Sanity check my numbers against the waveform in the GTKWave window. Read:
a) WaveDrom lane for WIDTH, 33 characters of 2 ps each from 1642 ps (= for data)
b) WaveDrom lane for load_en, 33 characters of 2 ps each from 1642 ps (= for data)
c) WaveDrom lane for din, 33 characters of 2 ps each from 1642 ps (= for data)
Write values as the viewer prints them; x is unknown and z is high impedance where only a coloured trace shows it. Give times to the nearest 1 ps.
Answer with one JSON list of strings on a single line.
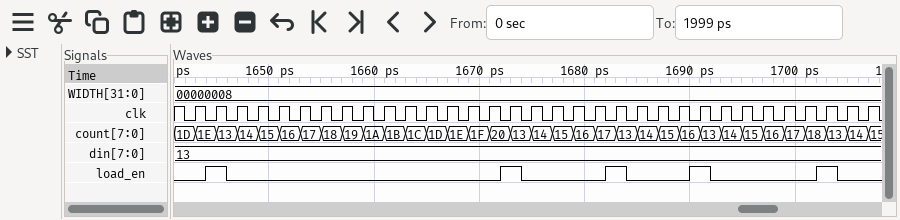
["{name: 'WIDTH', wave: '=................................', data: '00000008'}", "{name: 'load_en', wave: '010............10...10..10....10.'}", "{name: 'din', wave: '=................................', data: '13'}"]
